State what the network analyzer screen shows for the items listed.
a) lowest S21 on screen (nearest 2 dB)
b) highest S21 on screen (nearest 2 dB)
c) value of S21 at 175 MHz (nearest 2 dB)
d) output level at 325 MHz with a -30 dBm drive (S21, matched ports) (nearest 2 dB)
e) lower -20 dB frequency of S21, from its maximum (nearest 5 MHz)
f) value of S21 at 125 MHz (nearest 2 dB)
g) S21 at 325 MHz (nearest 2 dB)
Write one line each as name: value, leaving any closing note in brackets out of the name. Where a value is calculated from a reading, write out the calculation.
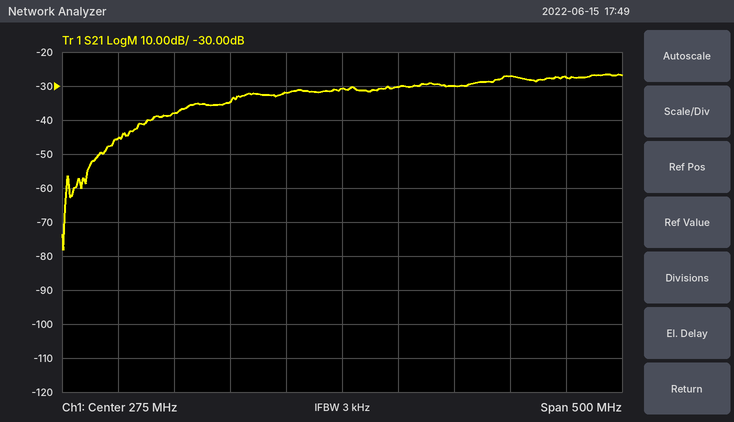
lowest S21 on screen: -78 dB
highest S21 on screen: -26 dB
value of S21 at 175 MHz: -34 dB
output level at 325 MHz with a -30 dBm drive (S21, matched ports): -30 dBm + (-30 dB) = -60 dBm
lower -20 dB frequency of S21, from its maximum: 70 MHz
value of S21 at 125 MHz: -38 dB
S21 at 325 MHz: -30 dB
